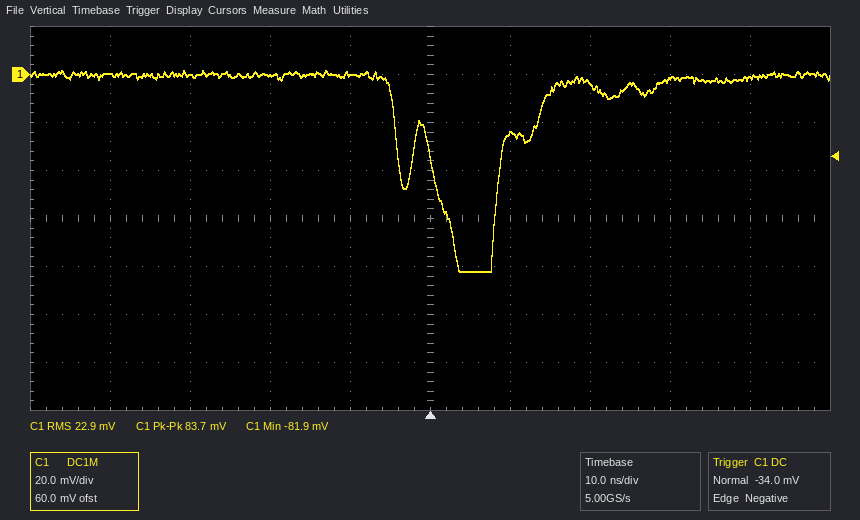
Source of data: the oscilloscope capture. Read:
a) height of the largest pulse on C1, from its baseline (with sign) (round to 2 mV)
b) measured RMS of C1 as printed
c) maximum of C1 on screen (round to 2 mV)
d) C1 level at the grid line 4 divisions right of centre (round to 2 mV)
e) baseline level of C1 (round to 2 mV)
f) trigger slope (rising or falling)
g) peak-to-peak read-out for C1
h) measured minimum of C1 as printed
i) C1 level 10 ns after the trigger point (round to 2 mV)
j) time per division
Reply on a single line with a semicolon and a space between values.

-82 mV; 22.9 mV; 2 mV; -2 mV; 0 mV; falling; 83.7 mV; -81.9 mV; -24 mV; 10 ns
